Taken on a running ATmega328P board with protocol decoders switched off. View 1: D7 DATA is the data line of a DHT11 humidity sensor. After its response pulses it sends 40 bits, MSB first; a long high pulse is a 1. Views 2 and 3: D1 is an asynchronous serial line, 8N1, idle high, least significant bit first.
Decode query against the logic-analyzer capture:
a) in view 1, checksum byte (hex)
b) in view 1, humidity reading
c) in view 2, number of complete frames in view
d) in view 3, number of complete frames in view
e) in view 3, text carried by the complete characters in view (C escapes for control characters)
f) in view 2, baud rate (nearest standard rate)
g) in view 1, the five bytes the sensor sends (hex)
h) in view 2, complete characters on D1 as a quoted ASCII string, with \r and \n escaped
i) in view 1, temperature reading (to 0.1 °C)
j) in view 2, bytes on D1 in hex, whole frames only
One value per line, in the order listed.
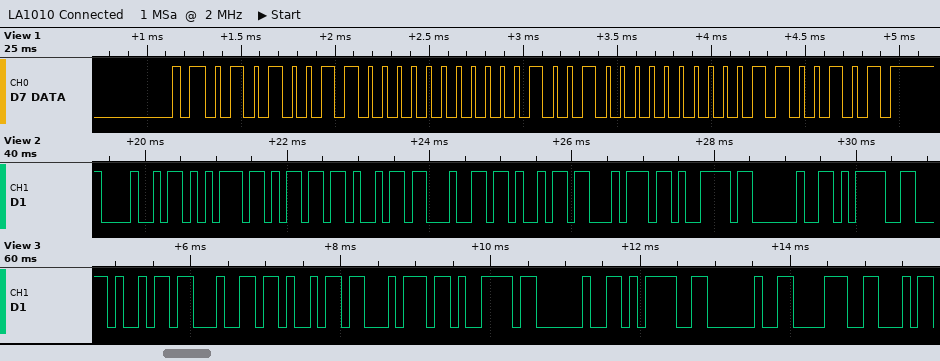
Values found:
0x65
83 %
10
9
"idity = 8"
9600 baud
53 00 12 00 65
"Humidity ="
18.0 °C
0x48 0x75 0x6D 0x69 0x64 0x69 0x74 0x79 0x20 0x3D
